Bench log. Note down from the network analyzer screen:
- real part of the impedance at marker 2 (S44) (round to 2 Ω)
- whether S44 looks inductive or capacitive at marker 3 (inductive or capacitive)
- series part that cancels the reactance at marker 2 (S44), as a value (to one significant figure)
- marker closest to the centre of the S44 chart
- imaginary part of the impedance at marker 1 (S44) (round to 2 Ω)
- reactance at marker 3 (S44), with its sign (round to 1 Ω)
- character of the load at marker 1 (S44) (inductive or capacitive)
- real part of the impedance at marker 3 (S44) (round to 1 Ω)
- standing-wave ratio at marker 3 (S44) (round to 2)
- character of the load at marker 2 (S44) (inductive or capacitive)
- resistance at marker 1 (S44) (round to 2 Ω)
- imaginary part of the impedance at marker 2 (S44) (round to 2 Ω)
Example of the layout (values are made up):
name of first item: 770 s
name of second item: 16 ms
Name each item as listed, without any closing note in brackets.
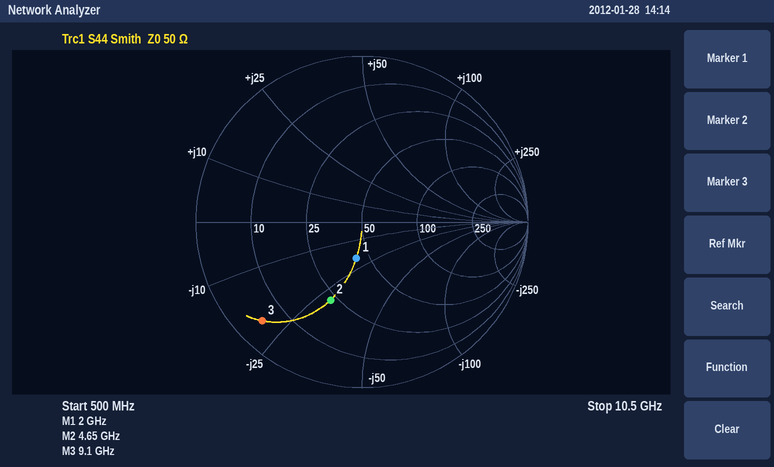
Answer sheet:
real part of the impedance at marker 2 (S44): 22 Ω
whether S44 looks inductive or capacitive at marker 3: capacitive
series part that cancels the reactance at marker 2 (S44), as a value: 1.0 nH
marker closest to the centre of the S44 chart: marker 1
imaginary part of the impedance at marker 1 (S44): -20 Ω
reactance at marker 3 (S44), with its sign: -20 Ω
character of the load at marker 1 (S44): capacitive
real part of the impedance at marker 3 (S44): 5 Ω
standing-wave ratio at marker 3 (S44): 12
character of the load at marker 2 (S44): capacitive
resistance at marker 1 (S44): 42 Ω
imaginary part of the impedance at marker 2 (S44): -28 Ω
